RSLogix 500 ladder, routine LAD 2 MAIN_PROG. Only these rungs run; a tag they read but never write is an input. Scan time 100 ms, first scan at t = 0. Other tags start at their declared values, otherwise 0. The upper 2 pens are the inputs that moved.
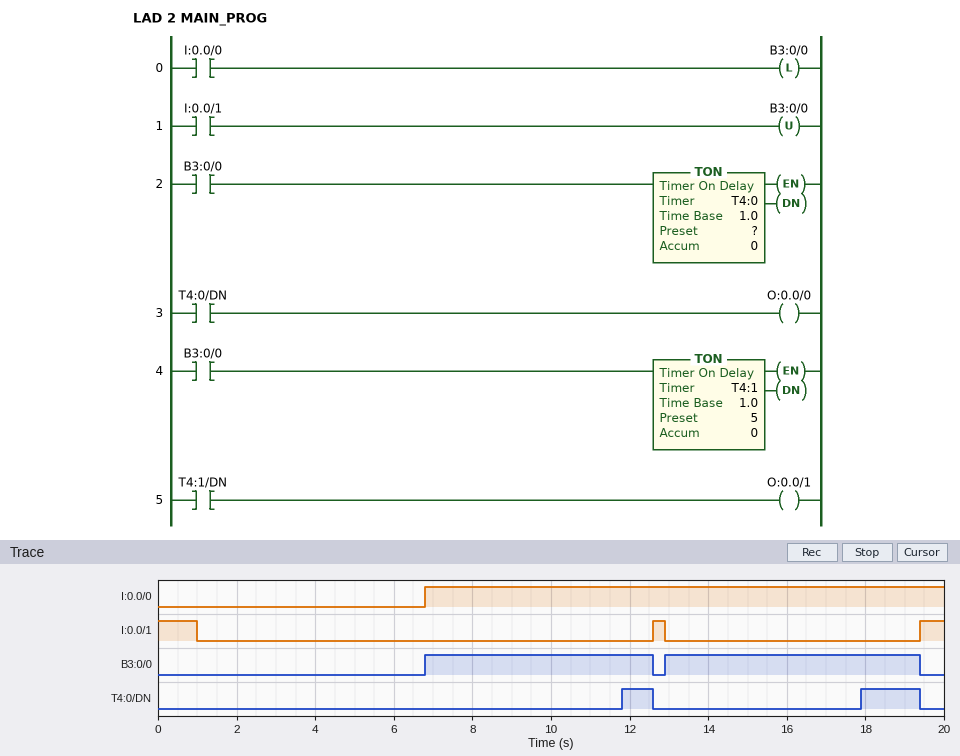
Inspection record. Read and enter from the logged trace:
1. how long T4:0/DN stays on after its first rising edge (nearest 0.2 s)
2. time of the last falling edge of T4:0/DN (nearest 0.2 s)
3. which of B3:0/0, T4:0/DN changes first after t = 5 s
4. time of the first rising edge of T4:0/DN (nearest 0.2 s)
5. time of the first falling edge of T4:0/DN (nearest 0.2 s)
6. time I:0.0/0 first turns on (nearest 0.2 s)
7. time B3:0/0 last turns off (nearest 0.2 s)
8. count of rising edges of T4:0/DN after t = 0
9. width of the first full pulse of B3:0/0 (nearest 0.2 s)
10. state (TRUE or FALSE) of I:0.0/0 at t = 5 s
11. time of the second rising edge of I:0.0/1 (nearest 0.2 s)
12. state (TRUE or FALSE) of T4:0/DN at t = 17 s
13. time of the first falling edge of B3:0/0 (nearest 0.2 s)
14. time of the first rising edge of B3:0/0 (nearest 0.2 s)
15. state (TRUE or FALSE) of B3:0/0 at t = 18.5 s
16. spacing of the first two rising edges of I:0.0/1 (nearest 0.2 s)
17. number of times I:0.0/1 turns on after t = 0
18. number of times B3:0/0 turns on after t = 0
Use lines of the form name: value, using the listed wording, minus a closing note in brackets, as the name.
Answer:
how long T4:0/DN stays on after its first rising edge: 0.8 s
time of the last falling edge of T4:0/DN: 19.4 s
which of B3:0/0, T4:0/DN changes first after t = 5 s: B3:0/0
time of the first rising edge of T4:0/DN: 11.8 s
time of the first falling edge of T4:0/DN: 12.6 s
time I:0.0/0 first turns on: 6.8 s
time B3:0/0 last turns off: 19.4 s
count of rising edges of T4:0/DN after t = 0: 2
width of the first full pulse of B3:0/0: 5.8 s
state (TRUE or FALSE) of I:0.0/0 at t = 5 s: FALSE
time of the second rising edge of I:0.0/1: 19.4 s
state (TRUE or FALSE) of T4:0/DN at t = 17 s: FALSE
time of the first falling edge of B3:0/0: 12.6 s
time of the first rising edge of B3:0/0: 6.8 s
state (TRUE or FALSE) of B3:0/0 at t = 18.5 s: TRUE
spacing of the first two rising edges of I:0.0/1: 6.8 s
number of times I:0.0/1 turns on after t = 0: 2
number of times B3:0/0 turns on after t = 0: 2
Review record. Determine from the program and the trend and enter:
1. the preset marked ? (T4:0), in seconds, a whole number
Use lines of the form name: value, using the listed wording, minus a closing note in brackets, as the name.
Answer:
the preset marked ? (T4:0), in seconds, a whole number: 5 s
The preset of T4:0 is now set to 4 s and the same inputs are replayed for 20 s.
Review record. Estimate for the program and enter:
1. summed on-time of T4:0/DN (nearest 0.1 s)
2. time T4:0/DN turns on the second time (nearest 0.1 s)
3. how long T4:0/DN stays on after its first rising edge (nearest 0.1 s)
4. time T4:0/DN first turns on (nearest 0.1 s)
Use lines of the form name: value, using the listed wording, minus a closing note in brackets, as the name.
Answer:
summed on-time of T4:0/DN: 4.3 s
time T4:0/DN turns on the second time: 16.9 s
how long T4:0/DN stays on after its first rising edge: 1.8 s
time T4:0/DN first turns on: 10.8 s
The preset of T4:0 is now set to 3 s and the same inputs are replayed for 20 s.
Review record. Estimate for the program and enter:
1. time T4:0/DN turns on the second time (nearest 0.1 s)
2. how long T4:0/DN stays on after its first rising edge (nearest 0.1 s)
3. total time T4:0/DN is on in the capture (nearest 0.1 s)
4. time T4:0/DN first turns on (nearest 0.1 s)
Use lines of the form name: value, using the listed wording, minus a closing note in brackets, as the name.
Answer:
time T4:0/DN turns on the second time: 15.9 s
how long T4:0/DN stays on after its first rising edge: 2.8 s
total time T4:0/DN is on in the capture: 6.3 s
time T4:0/DN first turns on: 9.8 s
